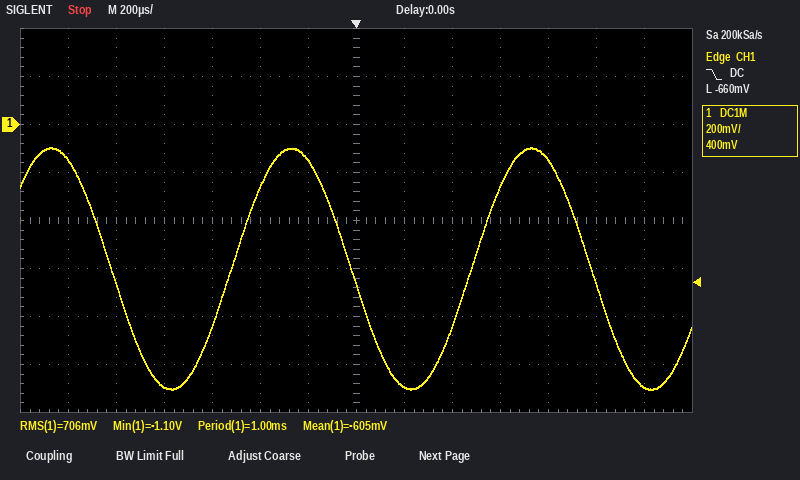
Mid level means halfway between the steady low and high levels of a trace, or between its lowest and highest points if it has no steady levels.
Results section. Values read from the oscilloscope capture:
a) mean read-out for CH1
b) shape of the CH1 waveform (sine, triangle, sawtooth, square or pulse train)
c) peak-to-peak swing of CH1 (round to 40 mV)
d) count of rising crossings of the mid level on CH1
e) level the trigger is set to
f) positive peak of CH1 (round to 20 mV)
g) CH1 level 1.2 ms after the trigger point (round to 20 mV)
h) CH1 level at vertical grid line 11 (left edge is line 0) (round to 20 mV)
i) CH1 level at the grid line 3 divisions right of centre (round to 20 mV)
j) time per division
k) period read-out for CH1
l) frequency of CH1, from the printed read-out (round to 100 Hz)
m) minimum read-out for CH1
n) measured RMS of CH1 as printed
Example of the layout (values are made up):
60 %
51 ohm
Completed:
-605 mV
sine
1.00 V
2
-660 mV
-100 mV
-1.10 V
-140 mV
-260 mV
200 µs
1.00 ms
1.0 kHz
-1.10 V
706 mV
